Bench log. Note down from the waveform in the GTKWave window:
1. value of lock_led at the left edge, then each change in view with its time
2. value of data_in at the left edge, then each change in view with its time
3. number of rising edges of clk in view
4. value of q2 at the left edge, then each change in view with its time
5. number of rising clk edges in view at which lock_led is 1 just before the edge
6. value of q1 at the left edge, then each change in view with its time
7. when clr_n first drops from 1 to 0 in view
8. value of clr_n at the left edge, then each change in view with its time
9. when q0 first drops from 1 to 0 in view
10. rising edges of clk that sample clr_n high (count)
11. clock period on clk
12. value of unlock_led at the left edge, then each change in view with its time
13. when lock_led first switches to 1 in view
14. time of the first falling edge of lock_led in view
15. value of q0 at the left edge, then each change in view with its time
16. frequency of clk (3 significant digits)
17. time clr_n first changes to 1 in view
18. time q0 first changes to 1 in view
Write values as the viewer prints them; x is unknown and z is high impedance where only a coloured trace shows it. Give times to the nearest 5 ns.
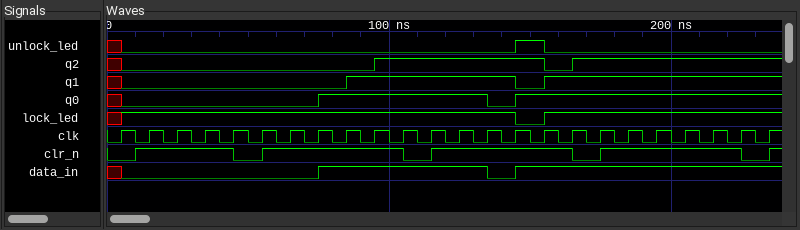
x, 1 at 5 ns, 0 at 145 ns, 1 at 155 ns
x, 0 at 5 ns, 1 at 75 ns, 0 at 135 ns, 1 at 145 ns
24
x, 0 at 5 ns, 1 at 95 ns, 0 at 155 ns, 1 at 165 ns
22
x, 0 at 5 ns, 1 at 85 ns, 0 at 145 ns, 1 at 155 ns
45 ns
0, 1 at 10 ns, 0 at 45 ns, 1 at 55 ns, 0 at 105 ns, 1 at 115 ns, 0 at 165 ns, 1 at 175 ns, 0 at 225 ns, 1 at 235 ns
135 ns
19
10 ns
x, 0 at 5 ns, 1 at 145 ns, 0 at 155 ns
5 ns
145 ns
x, 0 at 5 ns, 1 at 75 ns, 0 at 135 ns, 1 at 145 ns
100 MHz
10 ns
75 ns
